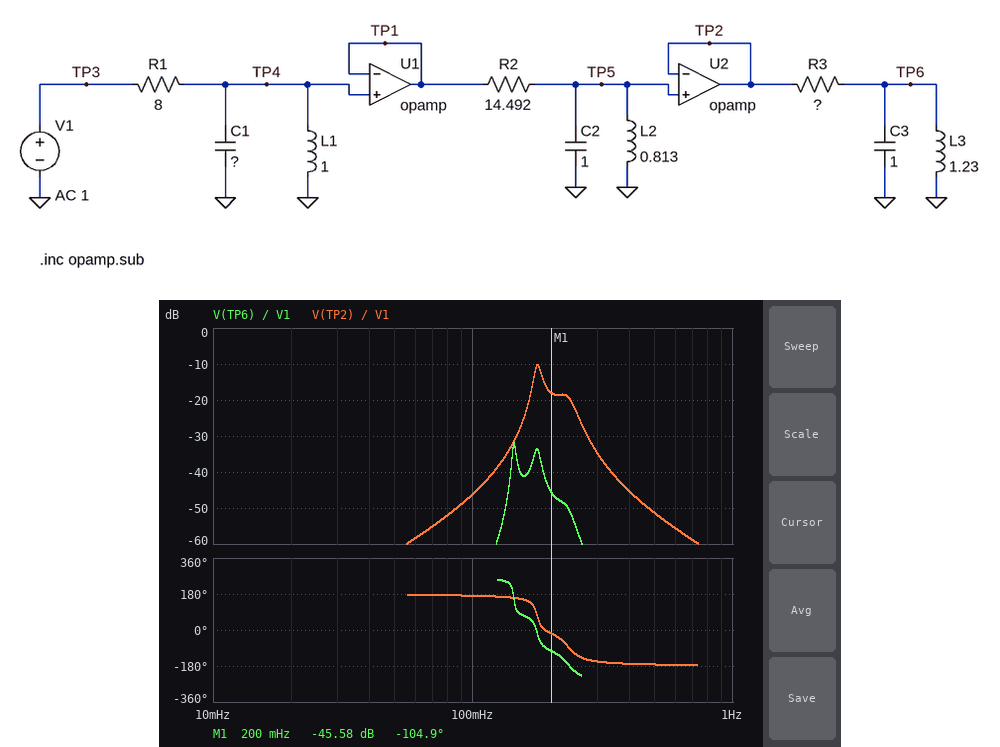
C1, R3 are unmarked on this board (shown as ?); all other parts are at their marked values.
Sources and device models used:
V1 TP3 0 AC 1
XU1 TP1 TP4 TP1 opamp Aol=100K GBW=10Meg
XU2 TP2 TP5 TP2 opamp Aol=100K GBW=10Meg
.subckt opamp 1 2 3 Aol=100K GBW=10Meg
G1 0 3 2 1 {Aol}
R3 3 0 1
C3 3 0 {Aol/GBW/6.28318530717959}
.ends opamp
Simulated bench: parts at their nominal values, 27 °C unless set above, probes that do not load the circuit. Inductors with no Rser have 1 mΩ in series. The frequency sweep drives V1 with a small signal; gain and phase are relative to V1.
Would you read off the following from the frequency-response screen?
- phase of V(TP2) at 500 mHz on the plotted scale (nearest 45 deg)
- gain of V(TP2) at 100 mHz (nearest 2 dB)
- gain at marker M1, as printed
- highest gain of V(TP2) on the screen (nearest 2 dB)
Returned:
-180 deg
-46 dB
-45.58 dB
-10 dB
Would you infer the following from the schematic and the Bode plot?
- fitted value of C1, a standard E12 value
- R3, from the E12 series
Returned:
470 mF
39 Ω
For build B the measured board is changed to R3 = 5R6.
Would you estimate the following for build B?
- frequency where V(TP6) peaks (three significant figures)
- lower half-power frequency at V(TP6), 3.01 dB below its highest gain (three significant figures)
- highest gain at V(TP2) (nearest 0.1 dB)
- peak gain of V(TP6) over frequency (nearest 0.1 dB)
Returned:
176 mHz
171 mHz
-10.2 dB
-17.6 dB
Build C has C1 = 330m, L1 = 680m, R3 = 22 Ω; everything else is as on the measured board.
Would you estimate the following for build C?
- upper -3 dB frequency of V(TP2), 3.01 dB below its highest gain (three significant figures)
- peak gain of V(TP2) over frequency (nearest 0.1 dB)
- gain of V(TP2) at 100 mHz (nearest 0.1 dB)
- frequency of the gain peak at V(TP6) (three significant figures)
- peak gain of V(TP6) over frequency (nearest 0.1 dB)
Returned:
183 mHz
-17.9 dB
-50.4 dB
176 mHz
-36.3 dB
